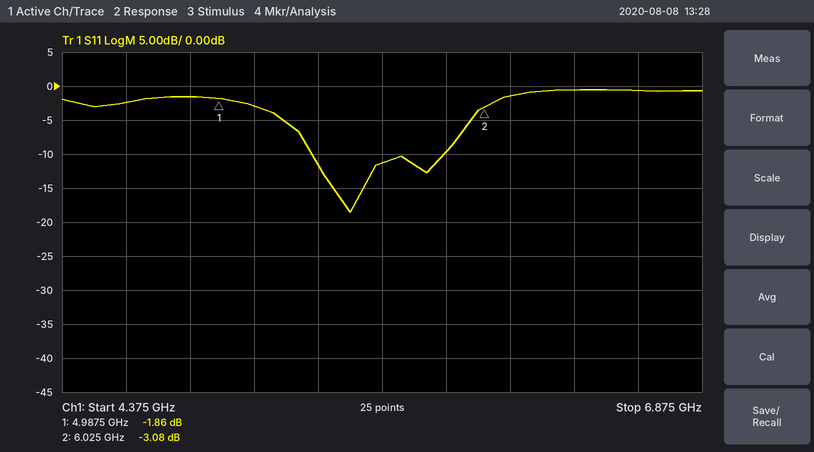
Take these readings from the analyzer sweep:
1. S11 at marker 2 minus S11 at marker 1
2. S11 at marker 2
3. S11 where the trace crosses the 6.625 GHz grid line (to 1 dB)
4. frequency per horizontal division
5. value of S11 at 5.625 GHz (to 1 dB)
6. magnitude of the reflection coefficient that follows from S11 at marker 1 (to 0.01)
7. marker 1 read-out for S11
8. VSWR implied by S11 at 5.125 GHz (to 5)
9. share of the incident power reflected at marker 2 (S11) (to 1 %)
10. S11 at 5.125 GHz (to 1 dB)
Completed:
-1.22 dB
-3.08 dB
-1 dB
250 MHz
-11 dB
0.81
-1.86 dB
5
49 %
-3 dB
